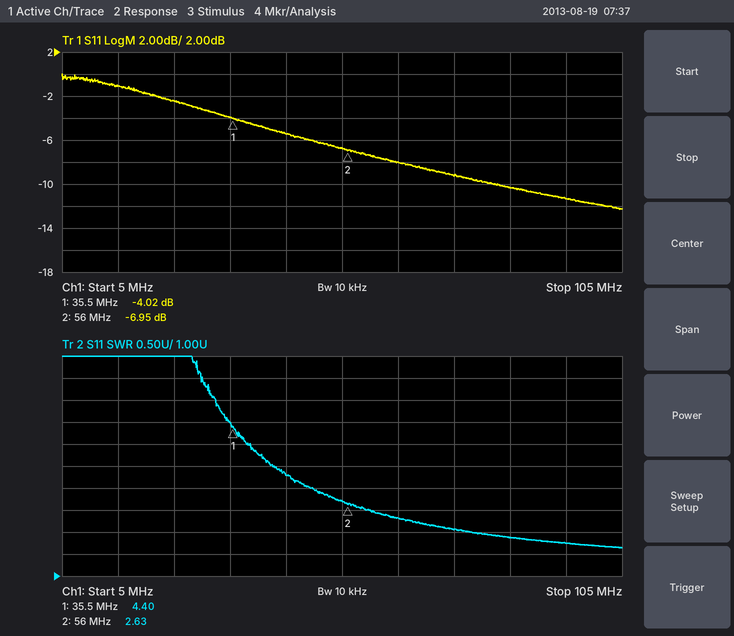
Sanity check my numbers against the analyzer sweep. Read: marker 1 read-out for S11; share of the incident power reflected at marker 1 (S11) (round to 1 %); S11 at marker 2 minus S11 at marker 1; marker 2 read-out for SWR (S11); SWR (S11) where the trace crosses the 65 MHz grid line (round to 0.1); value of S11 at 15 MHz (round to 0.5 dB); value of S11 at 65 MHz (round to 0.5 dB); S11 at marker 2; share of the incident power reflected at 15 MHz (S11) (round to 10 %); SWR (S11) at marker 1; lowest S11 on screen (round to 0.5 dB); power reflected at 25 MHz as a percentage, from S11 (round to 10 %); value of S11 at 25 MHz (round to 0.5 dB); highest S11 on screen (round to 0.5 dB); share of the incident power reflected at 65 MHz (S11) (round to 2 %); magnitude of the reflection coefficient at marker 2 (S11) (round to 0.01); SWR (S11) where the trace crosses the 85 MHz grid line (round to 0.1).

-4.02 dB
40 %
-2.93 dB
2.63
2.3
-1.0 dB
-8.0 dB
-6.95 dB
80 %
4.40
-12.5 dB
60 %
-2.5 dB
0.0 dB
16 %
0.45
1.9
